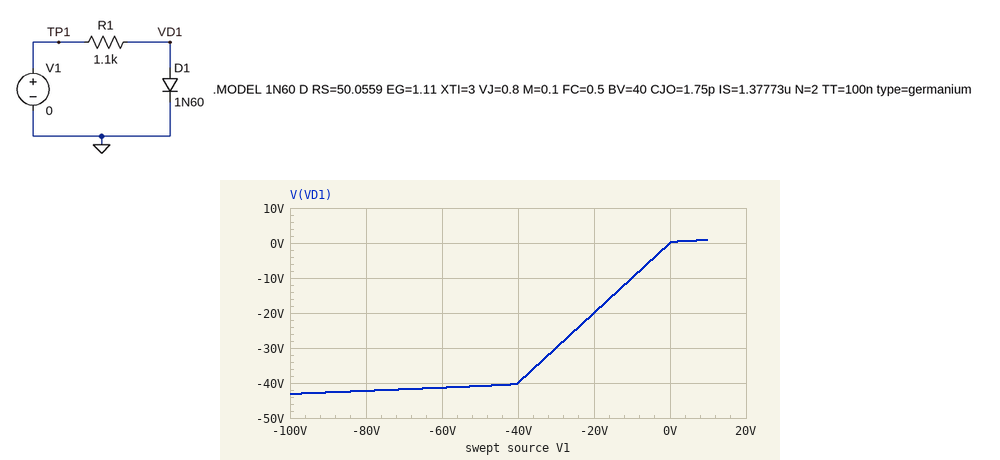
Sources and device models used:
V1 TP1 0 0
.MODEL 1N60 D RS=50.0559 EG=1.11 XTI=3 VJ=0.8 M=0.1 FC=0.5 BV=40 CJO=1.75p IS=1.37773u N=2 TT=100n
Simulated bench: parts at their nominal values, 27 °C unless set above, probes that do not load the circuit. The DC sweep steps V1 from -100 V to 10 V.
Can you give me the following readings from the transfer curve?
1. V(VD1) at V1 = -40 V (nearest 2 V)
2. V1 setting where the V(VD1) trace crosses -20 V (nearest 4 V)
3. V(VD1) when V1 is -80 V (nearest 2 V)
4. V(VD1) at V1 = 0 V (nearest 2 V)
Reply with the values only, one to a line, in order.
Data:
-40 V
-20 V
-42 V
0 V
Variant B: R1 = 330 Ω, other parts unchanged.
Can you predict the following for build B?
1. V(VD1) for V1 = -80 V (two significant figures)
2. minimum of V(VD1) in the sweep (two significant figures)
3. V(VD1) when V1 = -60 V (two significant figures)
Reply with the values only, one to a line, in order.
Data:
-46 V
-48 V
-43 V
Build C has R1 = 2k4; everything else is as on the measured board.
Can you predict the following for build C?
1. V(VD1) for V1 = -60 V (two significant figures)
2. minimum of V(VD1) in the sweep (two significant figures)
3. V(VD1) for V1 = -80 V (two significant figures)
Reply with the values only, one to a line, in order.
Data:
-41 V
-42 V
-41 V
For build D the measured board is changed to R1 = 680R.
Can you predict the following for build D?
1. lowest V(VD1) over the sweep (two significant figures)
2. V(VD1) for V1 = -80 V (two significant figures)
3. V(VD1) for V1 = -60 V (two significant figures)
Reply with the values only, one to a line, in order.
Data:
-45 V
-43 V
-42 V
